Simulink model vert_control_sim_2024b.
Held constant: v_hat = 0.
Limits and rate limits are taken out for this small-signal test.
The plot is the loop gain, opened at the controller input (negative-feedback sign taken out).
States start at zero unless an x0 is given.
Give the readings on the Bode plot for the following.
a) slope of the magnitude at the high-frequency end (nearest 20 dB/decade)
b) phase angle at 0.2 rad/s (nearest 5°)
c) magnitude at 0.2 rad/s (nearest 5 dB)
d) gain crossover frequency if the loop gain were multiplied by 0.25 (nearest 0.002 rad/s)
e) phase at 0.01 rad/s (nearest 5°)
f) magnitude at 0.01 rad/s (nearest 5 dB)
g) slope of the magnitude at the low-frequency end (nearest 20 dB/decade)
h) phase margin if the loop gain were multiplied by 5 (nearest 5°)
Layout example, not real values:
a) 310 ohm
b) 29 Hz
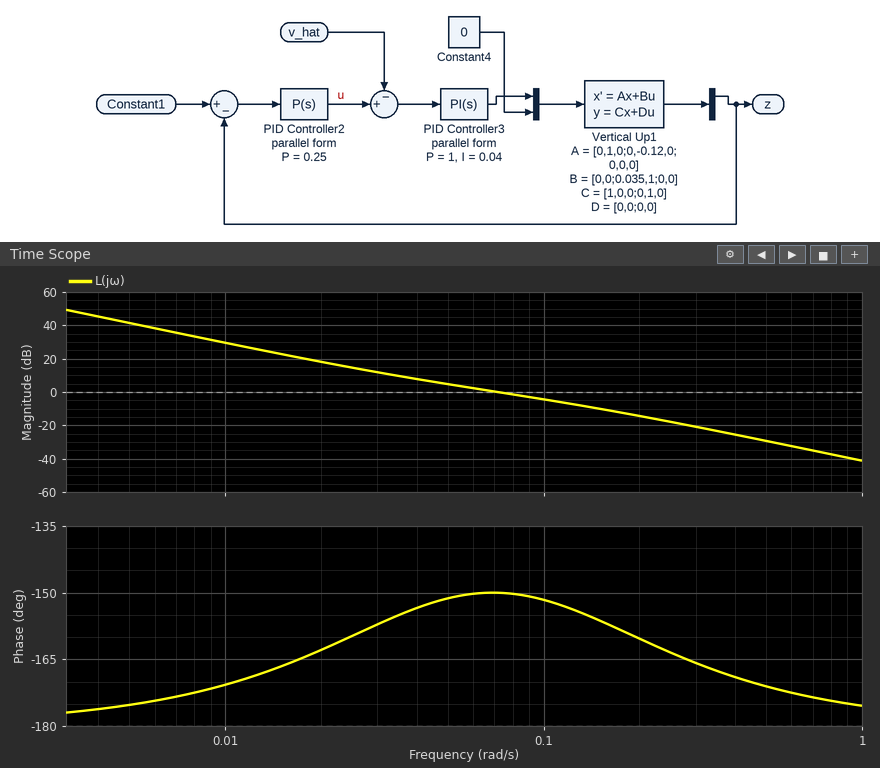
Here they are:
a) -40 dB/decade
b) -160°
c) -15 dB
d) 0.030 rad/s
e) -170°
f) 30 dB
g) -40 dB/decade
h) 20°
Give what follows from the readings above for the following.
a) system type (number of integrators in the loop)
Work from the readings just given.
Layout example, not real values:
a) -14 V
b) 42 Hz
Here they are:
a) 2
